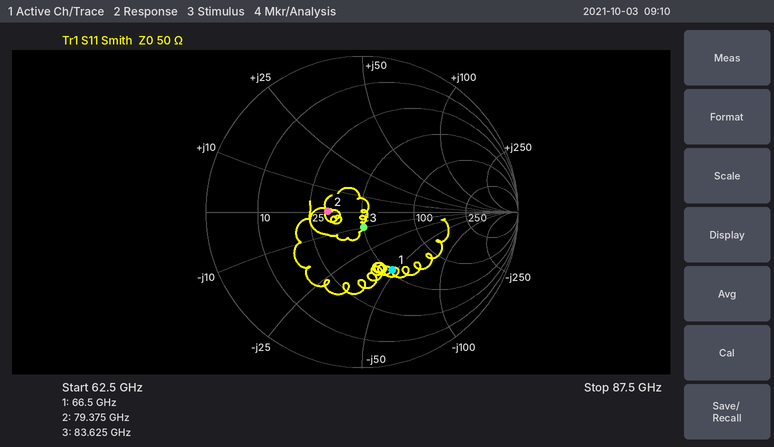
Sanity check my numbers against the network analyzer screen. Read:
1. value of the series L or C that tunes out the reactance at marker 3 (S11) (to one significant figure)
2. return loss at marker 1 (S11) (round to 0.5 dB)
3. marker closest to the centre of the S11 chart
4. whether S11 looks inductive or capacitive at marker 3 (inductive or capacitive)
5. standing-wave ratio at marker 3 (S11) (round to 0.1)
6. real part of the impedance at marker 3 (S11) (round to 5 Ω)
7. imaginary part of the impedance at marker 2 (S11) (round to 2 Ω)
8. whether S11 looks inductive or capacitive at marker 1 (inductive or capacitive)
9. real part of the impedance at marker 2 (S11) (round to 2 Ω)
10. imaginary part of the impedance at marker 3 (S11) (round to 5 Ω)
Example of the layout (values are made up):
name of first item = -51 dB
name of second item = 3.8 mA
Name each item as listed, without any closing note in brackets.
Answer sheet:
value of the series L or C that tunes out the reactance at marker 3 (S11) = 20 pH
return loss at marker 1 (S11) = 7.5 dB
marker closest to the centre of the S11 chart = marker 3
whether S11 looks inductive or capacitive at marker 3 = capacitive
standing-wave ratio at marker 3 (S11) = 1.2
real part of the impedance at marker 3 (S11) = 50 Ω
imaginary part of the impedance at marker 2 (S11) = 0 Ω
whether S11 looks inductive or capacitive at marker 1 = capacitive
real part of the impedance at marker 2 (S11) = 32 Ω
imaginary part of the impedance at marker 3 (S11) = -10 Ω
